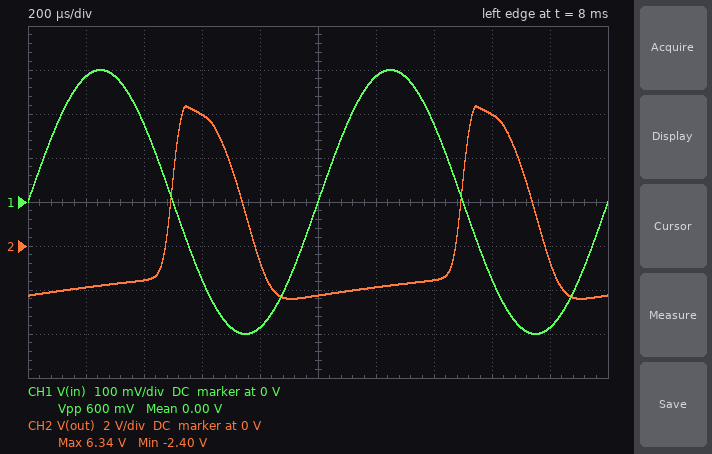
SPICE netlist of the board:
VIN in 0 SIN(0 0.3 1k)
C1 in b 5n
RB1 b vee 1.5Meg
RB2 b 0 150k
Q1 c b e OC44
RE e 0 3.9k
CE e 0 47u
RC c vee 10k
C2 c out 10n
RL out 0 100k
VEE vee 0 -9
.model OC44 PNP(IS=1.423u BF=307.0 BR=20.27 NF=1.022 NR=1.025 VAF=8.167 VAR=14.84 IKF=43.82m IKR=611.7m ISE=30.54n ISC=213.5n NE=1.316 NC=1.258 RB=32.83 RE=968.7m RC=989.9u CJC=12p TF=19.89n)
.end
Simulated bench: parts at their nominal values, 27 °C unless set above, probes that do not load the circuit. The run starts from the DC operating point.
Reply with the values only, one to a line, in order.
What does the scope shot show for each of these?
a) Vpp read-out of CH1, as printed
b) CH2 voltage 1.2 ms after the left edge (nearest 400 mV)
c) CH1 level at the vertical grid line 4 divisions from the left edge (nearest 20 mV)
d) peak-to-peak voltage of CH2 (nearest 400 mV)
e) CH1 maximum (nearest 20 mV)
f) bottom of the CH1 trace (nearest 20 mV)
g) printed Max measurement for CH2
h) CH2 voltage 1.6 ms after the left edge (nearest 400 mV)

600 mV
-2.0 V
-280 mV
8.8 V
300 mV
-300 mV
6.34 V
6.0 V
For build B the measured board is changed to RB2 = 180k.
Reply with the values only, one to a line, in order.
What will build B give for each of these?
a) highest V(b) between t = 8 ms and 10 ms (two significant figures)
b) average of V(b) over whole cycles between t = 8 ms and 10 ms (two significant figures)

-460 mV
-700 mV
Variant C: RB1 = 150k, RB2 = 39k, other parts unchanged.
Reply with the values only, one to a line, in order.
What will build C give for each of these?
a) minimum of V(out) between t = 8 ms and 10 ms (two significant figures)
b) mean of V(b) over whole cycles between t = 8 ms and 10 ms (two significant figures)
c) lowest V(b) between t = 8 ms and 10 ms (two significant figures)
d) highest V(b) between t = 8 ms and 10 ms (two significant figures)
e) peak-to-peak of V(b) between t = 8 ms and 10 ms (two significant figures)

-3.5 V
-1.7 V
-1.8 V
-1.6 V
170 mV
